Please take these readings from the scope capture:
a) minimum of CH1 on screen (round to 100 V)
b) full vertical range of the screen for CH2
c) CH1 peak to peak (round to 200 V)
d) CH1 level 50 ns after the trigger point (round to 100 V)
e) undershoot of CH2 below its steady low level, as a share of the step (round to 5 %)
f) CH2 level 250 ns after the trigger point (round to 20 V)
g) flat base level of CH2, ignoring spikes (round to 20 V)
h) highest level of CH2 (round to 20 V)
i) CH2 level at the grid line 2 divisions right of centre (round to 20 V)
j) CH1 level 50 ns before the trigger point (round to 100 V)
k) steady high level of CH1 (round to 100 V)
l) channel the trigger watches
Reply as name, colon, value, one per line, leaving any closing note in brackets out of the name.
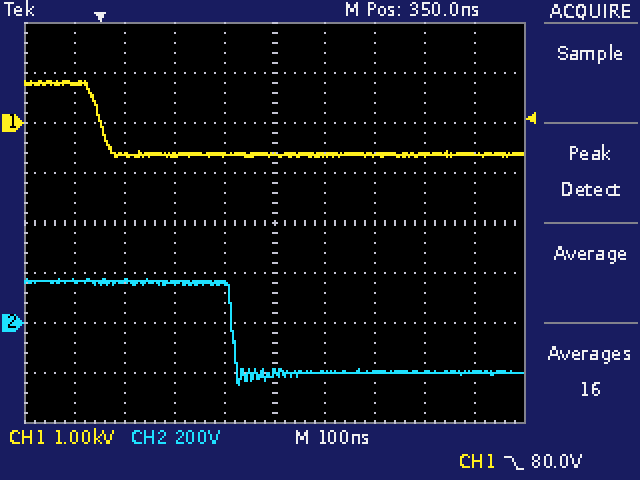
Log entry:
minimum of CH1 on screen: -700 V
full vertical range of the screen for CH2: 1.6 kV
CH1 peak to peak: 1.6 kV
CH1 level 50 ns after the trigger point: -600 V
undershoot of CH2 below its steady low level, as a share of the step: 15 %
CH2 level 250 ns after the trigger point: 160 V
flat base level of CH2, ignoring spikes: -200 V
highest level of CH2: 180 V
CH2 level at the grid line 2 divisions right of centre: -200 V
CH1 level 50 ns before the trigger point: 800 V
steady high level of CH1: 800 V
channel the trigger watches: CH1
